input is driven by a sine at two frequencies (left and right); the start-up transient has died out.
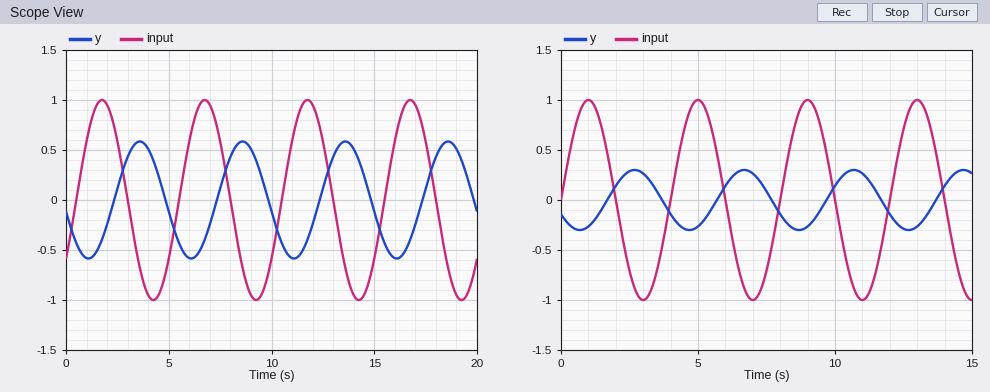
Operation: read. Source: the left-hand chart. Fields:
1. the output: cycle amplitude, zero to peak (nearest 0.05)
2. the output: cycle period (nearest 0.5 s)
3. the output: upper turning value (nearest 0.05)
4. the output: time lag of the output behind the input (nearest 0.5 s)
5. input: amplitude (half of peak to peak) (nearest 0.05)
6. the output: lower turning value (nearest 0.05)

0.60
5.0 s
0.60
2.0 s
1.00
-0.60
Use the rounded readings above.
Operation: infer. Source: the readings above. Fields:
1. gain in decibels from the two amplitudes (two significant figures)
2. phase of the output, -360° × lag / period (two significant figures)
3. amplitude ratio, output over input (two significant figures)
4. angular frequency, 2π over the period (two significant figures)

-4.4 dB
-140°
0.60
1.3 rad/s
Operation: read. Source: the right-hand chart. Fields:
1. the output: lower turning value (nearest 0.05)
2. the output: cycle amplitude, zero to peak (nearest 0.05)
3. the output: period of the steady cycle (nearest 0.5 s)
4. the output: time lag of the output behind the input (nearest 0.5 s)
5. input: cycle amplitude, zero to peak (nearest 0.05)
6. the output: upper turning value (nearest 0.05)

-0.30
0.30
4.0 s
1.5 s
1.00
0.30
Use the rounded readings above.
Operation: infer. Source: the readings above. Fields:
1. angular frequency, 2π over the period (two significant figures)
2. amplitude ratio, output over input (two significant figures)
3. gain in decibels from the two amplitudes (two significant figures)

1.6 rad/s
0.30
-10 dB
